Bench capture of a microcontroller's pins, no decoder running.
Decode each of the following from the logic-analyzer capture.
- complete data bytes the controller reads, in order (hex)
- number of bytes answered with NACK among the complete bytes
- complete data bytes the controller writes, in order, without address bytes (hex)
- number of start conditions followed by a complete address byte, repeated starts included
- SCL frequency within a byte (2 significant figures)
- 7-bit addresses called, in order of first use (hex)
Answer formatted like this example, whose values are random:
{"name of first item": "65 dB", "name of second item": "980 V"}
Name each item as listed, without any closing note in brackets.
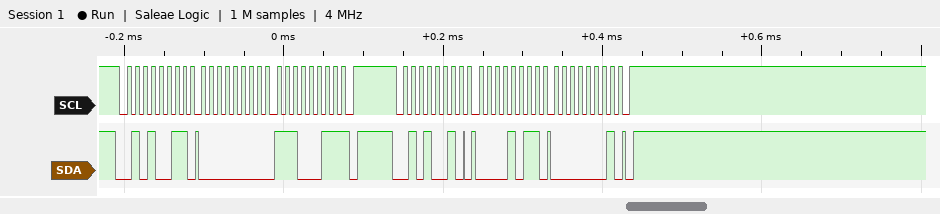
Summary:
{"complete data bytes the controller reads, in order": "00 E3", "number of bytes answered with NACK among the complete bytes": "1", "complete data bytes the controller writes, in order, without address bytes": "0B 01", "number of start conditions followed by a complete address byte, repeated starts included": "2", "SCL frequency within a byte": "100 kHz", "7-bit addresses called, in order of first use": "0x29"}
